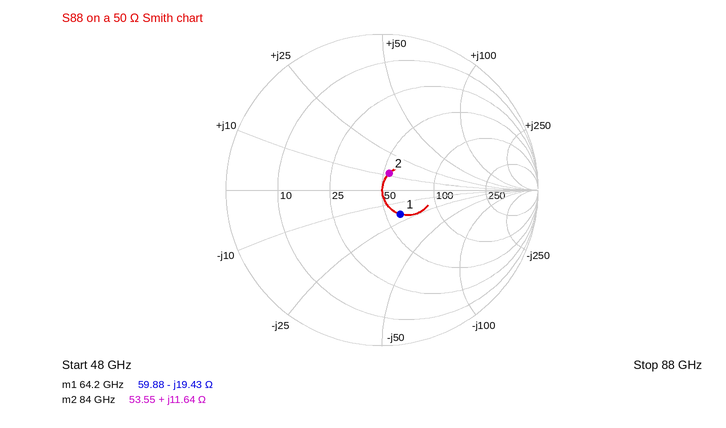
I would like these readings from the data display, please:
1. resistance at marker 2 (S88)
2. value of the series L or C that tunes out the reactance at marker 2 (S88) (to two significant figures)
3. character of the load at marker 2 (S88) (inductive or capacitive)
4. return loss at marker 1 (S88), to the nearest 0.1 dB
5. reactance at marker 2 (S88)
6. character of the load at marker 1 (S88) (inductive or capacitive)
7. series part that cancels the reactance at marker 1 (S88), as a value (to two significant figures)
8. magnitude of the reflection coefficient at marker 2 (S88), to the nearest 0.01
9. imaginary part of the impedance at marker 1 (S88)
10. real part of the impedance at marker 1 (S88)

53.55 Ω
160 fF
inductive
14.2 dB
+11.64 Ω
capacitive
48 pH
0.12
-19.43 Ω
59.88 Ω
